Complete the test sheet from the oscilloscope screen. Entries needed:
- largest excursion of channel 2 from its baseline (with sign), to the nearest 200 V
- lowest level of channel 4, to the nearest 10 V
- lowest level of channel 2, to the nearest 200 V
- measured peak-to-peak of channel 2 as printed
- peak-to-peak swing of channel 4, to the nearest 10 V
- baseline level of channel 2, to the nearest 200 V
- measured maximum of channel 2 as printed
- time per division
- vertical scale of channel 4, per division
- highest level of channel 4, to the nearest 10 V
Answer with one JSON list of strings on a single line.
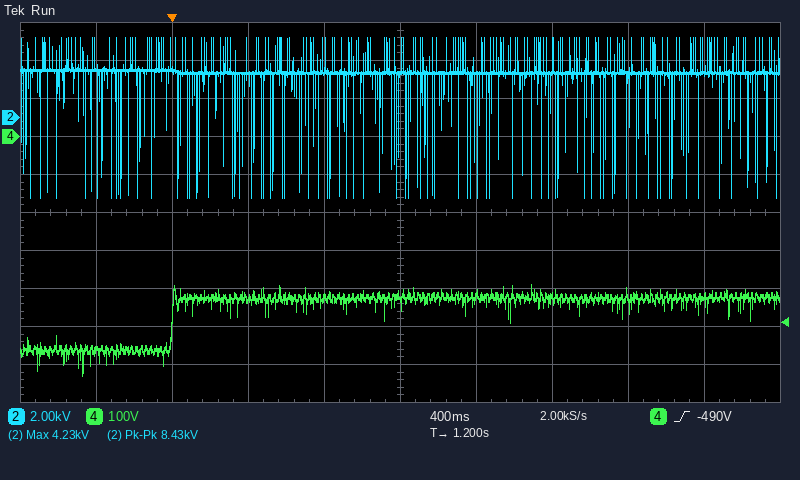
["-6.6 kV", "-630 V", "-4.2 kV", "8.43 kV", "240 V", "2.4 kV", "4.23 kV", "400 ms", "100 V", "-390 V"]
